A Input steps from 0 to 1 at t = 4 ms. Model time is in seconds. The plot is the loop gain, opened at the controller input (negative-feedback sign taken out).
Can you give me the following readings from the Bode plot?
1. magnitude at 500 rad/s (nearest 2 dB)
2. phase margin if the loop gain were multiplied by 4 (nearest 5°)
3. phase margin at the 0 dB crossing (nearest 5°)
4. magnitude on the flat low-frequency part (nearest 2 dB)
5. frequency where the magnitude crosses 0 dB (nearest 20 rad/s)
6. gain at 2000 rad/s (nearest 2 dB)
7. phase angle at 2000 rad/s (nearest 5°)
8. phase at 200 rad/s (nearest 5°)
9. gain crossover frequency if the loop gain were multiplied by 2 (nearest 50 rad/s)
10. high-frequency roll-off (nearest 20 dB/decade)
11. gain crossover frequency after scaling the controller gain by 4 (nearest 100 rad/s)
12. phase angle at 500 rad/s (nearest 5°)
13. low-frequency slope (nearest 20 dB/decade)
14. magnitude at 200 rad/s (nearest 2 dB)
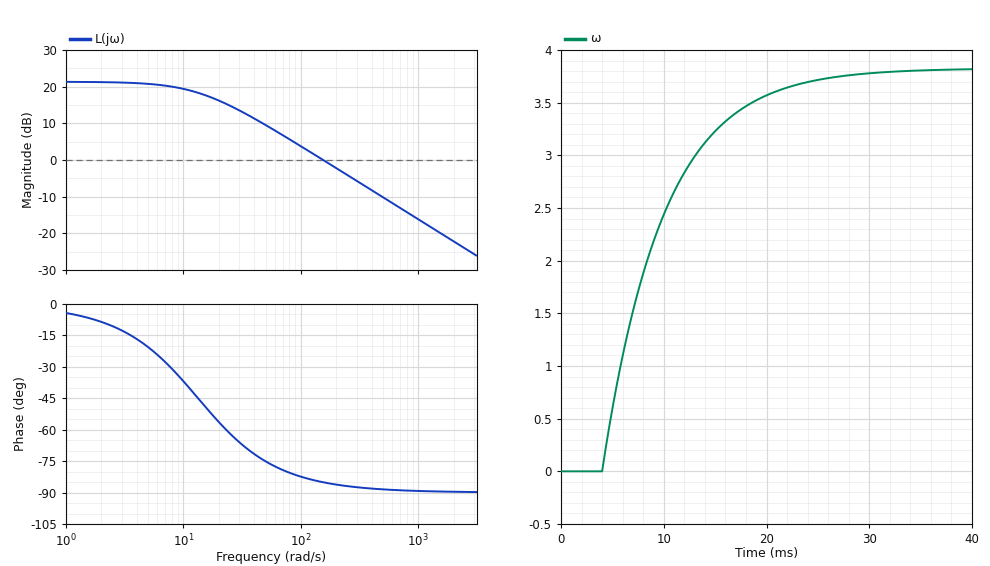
-10 dB
90°
95°
22 dB
160 rad/s
-22 dB
-90°
-85°
300 rad/s
-20 dB/decade
600 rad/s
-90°
0 dB/decade
-2 dB
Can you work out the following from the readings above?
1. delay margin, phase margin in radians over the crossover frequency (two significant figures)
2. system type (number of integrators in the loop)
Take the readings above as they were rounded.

0.010 s
0
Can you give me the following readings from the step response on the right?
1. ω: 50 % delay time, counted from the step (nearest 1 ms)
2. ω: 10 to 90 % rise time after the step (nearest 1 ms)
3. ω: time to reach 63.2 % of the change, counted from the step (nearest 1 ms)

4 ms
13 ms
6 ms
